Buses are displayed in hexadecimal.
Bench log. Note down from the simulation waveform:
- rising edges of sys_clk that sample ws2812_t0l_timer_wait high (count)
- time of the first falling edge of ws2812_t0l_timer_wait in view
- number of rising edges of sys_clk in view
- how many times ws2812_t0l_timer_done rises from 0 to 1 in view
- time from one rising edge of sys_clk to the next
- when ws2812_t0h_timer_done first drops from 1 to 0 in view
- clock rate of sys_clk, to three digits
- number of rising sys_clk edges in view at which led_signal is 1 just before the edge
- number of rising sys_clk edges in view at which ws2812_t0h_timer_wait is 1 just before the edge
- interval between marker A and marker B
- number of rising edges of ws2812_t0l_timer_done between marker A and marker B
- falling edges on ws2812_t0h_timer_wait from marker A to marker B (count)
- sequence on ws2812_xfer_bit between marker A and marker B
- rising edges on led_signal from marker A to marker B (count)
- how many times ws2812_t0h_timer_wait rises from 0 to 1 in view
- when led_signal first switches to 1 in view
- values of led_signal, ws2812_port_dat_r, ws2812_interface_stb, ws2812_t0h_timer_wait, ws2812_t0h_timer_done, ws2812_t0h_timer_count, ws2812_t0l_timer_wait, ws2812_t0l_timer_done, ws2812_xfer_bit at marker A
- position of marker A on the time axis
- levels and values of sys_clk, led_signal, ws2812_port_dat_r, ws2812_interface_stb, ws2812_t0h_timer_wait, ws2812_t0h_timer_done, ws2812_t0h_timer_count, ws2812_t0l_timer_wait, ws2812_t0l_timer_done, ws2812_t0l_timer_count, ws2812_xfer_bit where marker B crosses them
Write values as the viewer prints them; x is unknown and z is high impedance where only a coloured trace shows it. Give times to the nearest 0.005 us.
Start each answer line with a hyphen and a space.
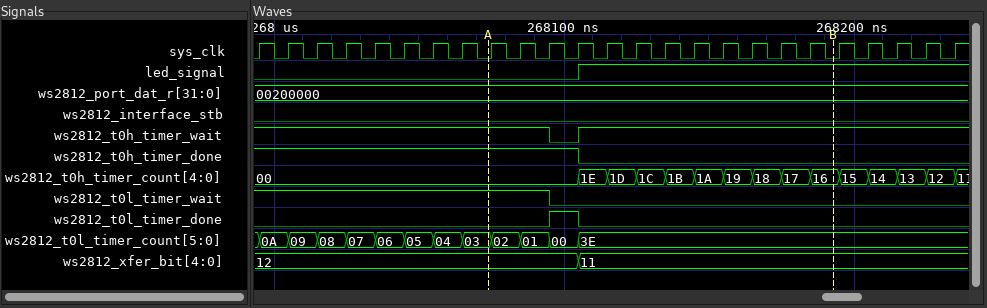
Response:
- 11
- 268.095 us
- 25
- 1
- 0.01 us
- 268.105 us
- 100 MHz
- 13
- 24
- 0.12 us
- 1
- 1
- 12, 11
- 1
- 1
- 268.105 us
- led_signal=0, ws2812_port_dat_r=00200000, ws2812_interface_stb=0, ws2812_t0h_timer_wait=1, ws2812_t0h_timer_done=1, ws2812_t0h_timer_count=00, ws2812_t0l_timer_wait=1, ws2812_t0l_timer_done=0, ws2812_xfer_bit=12
- 268.075 us
- sys_clk=0, led_signal=1, ws2812_port_dat_r=00200000, ws2812_interface_stb=0, ws2812_t0h_timer_wait=1, ws2812_t0h_timer_done=0, ws2812_t0h_timer_count=16, ws2812_t0l_timer_wait=0, ws2812_t0l_timer_done=0, ws2812_t0l_timer_count=3E, ws2812_xfer_bit=11
